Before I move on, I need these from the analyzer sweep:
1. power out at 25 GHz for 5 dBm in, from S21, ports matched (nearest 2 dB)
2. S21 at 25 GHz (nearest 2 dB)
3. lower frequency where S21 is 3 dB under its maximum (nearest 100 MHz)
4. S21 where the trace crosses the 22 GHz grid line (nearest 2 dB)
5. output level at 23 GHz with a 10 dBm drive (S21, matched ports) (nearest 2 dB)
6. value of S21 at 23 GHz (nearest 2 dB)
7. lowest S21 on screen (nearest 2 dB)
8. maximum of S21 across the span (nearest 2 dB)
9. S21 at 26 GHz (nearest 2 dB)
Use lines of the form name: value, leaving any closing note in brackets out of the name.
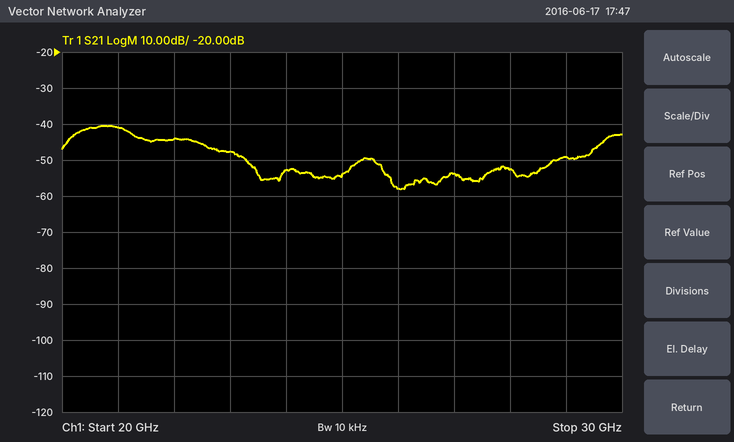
power out at 25 GHz for 5 dBm in, from S21, ports matched: -50 dBm
S21 at 25 GHz: -54 dB
lower frequency where S21 is 3 dB under its maximum: 20.2 GHz
S21 where the trace crosses the 22 GHz grid line: -44 dB
output level at 23 GHz with a 10 dBm drive (S21, matched ports): -38 dBm
value of S21 at 23 GHz: -48 dB
lowest S21 on screen: -58 dB
maximum of S21 across the span: -40 dB
S21 at 26 GHz: -58 dB
